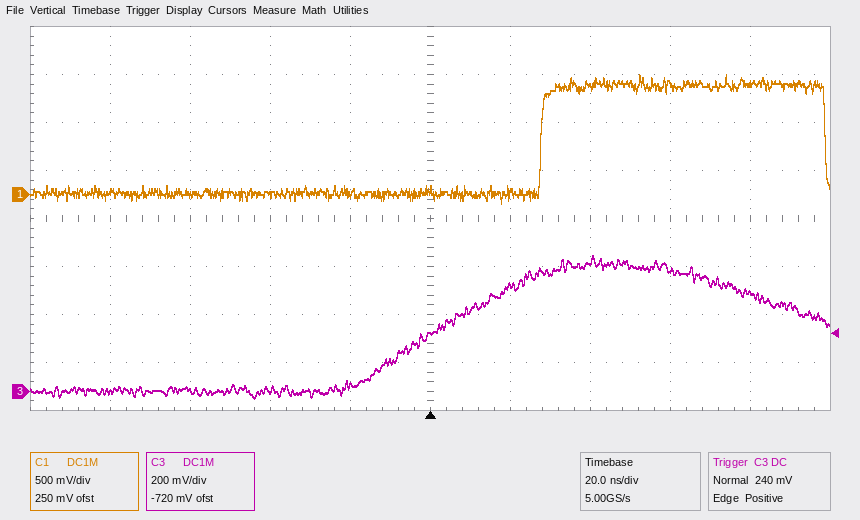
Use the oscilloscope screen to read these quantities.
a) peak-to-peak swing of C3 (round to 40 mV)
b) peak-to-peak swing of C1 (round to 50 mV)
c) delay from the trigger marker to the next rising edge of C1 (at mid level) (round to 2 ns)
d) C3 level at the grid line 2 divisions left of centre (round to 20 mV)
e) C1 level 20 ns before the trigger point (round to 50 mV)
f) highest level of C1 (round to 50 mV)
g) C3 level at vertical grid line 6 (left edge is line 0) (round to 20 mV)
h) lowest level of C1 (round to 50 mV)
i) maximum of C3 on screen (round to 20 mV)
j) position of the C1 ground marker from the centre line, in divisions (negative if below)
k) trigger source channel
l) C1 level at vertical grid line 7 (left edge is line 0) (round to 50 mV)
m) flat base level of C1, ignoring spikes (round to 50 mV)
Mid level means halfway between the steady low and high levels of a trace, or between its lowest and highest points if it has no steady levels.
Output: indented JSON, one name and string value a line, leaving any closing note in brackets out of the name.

{
  "peak-to-peak swing of C3": "600 mV",
  "peak-to-peak swing of C1": "1.35 V",
  "delay from the trigger marker to the next rising edge of C1 (at mid level)": "28 ns",
  "C3 level at the grid line 2 divisions left of centre": "0 mV",
  "C1 level 20 ns before the trigger point": "0 mV",
  "highest level of C1": "1.25 V",
  "C3 level at vertical grid line 6 (left edge is line 0)": "440 mV",
  "lowest level of C1": "-100 mV",
  "maximum of C3 on screen": "560 mV",
  "position of the C1 ground marker from the centre line, in divisions": "+0.5 div",
  "trigger source channel": "C3",
  "C1 level at vertical grid line 7 (left edge is line 0)": "1.15 V",
  "flat base level of C1, ignoring spikes": "0 mV"
}
